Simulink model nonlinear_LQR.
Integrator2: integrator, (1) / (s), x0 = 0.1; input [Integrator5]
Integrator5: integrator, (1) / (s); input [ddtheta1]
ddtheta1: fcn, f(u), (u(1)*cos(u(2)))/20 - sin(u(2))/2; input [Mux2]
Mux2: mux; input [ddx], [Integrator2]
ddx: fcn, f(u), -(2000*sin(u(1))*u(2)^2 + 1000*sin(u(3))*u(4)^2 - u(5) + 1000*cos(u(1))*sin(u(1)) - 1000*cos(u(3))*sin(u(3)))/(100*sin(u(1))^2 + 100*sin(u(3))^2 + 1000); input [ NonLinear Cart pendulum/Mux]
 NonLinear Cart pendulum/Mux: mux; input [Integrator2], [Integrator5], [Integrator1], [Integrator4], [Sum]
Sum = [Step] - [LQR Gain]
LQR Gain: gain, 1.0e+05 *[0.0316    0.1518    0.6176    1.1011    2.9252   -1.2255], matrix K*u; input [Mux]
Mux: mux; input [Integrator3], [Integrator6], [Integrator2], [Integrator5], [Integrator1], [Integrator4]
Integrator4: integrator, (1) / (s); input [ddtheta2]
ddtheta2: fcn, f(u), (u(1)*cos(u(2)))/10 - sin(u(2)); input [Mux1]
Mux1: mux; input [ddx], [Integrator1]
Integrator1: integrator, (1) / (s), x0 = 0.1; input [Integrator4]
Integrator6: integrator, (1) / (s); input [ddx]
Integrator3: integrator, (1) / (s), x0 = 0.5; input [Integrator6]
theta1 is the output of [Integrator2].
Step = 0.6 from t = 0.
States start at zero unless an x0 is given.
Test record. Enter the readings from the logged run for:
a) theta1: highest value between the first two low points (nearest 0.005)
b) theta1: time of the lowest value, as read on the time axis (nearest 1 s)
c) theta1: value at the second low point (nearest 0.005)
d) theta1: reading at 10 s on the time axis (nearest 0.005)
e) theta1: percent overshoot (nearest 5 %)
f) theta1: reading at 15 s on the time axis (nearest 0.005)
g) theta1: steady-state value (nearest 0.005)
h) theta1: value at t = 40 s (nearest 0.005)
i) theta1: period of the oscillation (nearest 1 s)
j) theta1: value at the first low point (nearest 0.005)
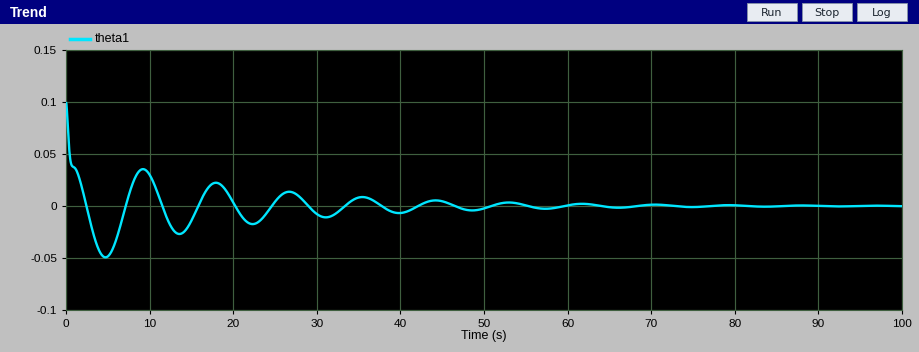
0.035
5 s
-0.025
0.030
50 %
-0.015
0.000
-0.005
9 s
-0.050
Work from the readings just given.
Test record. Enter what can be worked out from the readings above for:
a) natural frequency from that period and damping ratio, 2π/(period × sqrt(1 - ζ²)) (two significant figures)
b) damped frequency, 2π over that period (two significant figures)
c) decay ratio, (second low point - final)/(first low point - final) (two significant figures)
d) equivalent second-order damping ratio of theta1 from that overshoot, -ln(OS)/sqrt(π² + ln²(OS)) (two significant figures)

0.72 rad/s
0.70 rad/s
0.50
0.22
